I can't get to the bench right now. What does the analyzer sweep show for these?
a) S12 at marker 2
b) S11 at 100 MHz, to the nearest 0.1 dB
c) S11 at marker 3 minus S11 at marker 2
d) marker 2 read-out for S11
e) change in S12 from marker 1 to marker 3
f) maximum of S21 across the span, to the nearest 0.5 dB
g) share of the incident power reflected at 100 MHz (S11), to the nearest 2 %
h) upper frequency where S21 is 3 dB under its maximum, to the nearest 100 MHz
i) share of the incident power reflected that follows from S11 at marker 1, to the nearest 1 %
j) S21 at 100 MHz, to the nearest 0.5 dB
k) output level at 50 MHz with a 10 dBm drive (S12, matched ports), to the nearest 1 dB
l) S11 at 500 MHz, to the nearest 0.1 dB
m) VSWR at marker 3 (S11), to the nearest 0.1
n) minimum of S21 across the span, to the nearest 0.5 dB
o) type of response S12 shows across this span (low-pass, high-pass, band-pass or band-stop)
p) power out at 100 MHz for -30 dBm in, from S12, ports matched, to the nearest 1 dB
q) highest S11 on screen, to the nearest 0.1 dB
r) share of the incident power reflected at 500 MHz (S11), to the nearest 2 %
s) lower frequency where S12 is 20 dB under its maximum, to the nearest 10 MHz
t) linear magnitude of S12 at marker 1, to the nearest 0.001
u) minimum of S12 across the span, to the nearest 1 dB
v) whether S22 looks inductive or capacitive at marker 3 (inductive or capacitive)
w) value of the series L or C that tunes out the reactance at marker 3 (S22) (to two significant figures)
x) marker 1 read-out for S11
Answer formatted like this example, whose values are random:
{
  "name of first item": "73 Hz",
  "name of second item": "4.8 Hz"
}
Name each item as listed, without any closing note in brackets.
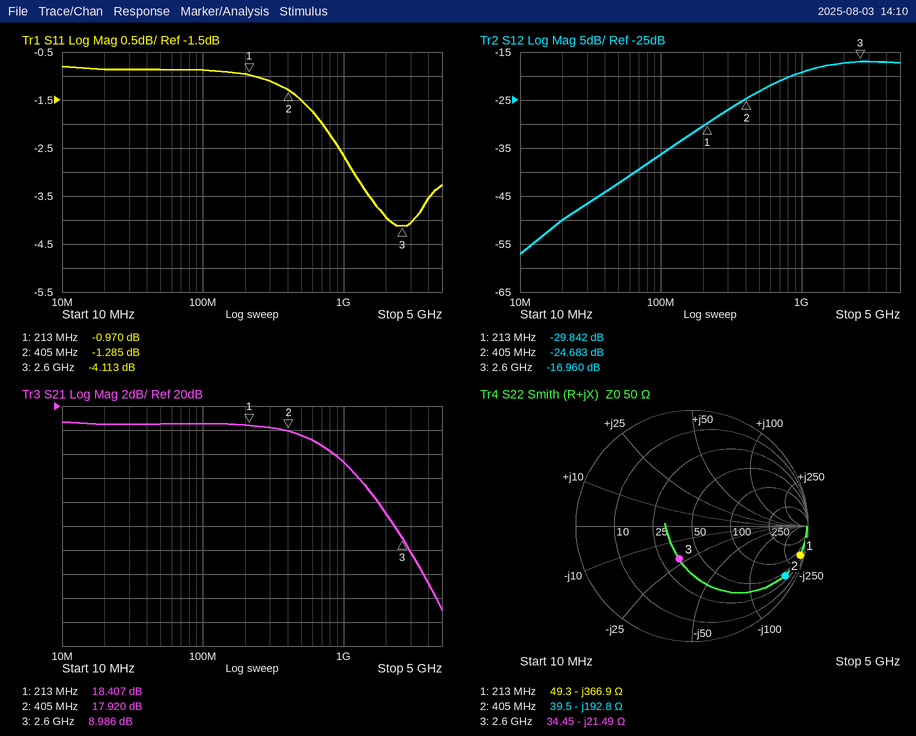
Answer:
{
  "S12 at marker 2": "-24.683 dB",
  "S11 at 100 MHz, to the nearest 0.1 dB": "-0.9 dB",
  "S11 at marker 3 minus S11 at marker 2": "-2.828 dB",
  "marker 2 read-out for S11": "-1.285 dB",
  "change in S12 from marker 1 to marker 3": "12.882 dB",
  "maximum of S21 across the span, to the nearest 0.5 dB": "18.5 dB",
  "share of the incident power reflected at 100 MHz (S11), to the nearest 2 %": "82 %",
  "upper frequency where S21 is 3 dB under its maximum, to the nearest 100 MHz": "900 MHz",
  "share of the incident power reflected that follows from S11 at marker 1, to the nearest 1 %": "80 %",
  "S21 at 100 MHz, to the nearest 0.5 dB": "18.5 dB",
  "output level at 50 MHz with a 10 dBm drive (S12, matched ports), to the nearest 1 dB": "-32 dBm",
  "S11 at 500 MHz, to the nearest 0.1 dB": "-1.5 dB",
  "VSWR at marker 3 (S11), to the nearest 0.1": "4.3",
  "minimum of S21 across the span, to the nearest 0.5 dB": "3.0 dB",
  "type of response S12 shows across this span": "high-pass",
  "power out at 100 MHz for -30 dBm in, from S12, ports matched, to the nearest 1 dB": "-66 dBm",
  "highest S11 on screen, to the nearest 0.1 dB": "-0.8 dB",
  "share of the incident power reflected at 500 MHz (S11), to the nearest 2 %": "70 %",
  "lower frequency where S12 is 20 dB under its maximum, to the nearest 10 MHz": "90 MHz",
  "linear magnitude of S12 at marker 1, to the nearest 0.001": "0.032",
  "minimum of S12 across the span, to the nearest 1 dB": "-57 dB",
  "whether S22 looks inductive or capacitive at marker 3": "capacitive",
  "value of the series L or C that tunes out the reactance at marker 3 (S22)": "1.3 nH",
  "marker 1 read-out for S11": "-0.970 dB"
}
